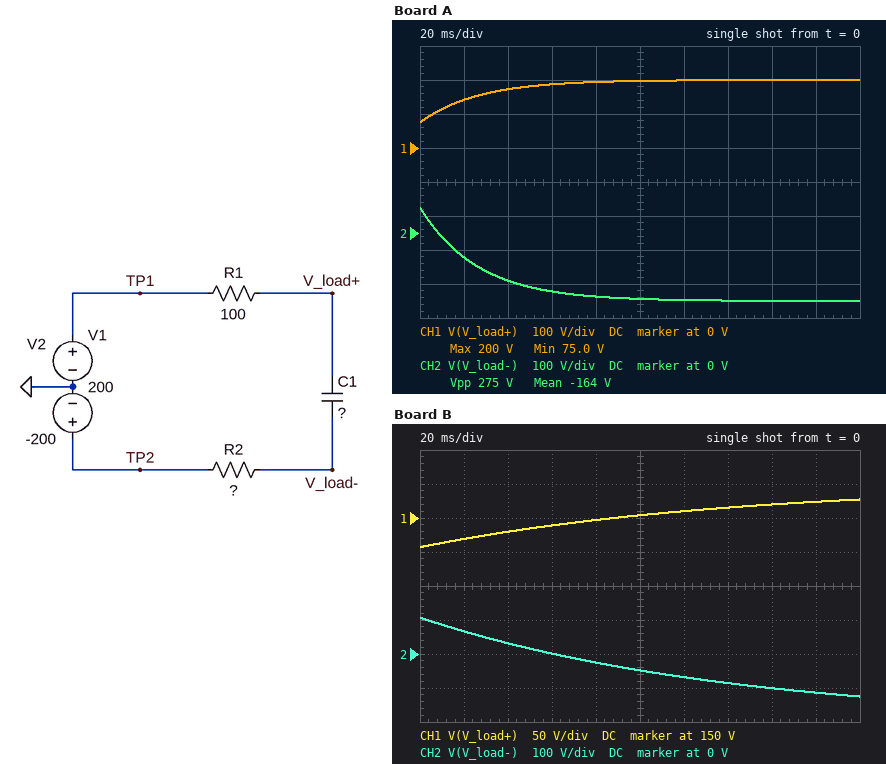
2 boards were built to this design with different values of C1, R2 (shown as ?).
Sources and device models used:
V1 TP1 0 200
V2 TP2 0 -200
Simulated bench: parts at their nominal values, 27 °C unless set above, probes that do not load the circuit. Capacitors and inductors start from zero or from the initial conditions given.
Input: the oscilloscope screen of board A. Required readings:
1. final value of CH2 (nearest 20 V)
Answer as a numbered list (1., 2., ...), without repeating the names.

1. -200 V
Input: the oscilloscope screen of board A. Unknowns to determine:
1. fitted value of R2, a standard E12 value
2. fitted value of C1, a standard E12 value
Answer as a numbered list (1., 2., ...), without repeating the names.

1. 220 Ω
2. 82 µF
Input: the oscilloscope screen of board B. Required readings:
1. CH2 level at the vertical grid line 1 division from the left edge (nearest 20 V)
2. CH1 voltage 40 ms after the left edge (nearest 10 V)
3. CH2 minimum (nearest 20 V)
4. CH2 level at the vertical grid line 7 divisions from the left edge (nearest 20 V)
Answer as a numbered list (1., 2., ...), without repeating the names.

1. 60 V
2. 130 V
3. -120 V
4. -80 V
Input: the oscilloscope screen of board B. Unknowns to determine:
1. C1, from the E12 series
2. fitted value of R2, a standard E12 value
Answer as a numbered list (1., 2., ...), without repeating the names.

1. 330 µF
2. 330 Ω
